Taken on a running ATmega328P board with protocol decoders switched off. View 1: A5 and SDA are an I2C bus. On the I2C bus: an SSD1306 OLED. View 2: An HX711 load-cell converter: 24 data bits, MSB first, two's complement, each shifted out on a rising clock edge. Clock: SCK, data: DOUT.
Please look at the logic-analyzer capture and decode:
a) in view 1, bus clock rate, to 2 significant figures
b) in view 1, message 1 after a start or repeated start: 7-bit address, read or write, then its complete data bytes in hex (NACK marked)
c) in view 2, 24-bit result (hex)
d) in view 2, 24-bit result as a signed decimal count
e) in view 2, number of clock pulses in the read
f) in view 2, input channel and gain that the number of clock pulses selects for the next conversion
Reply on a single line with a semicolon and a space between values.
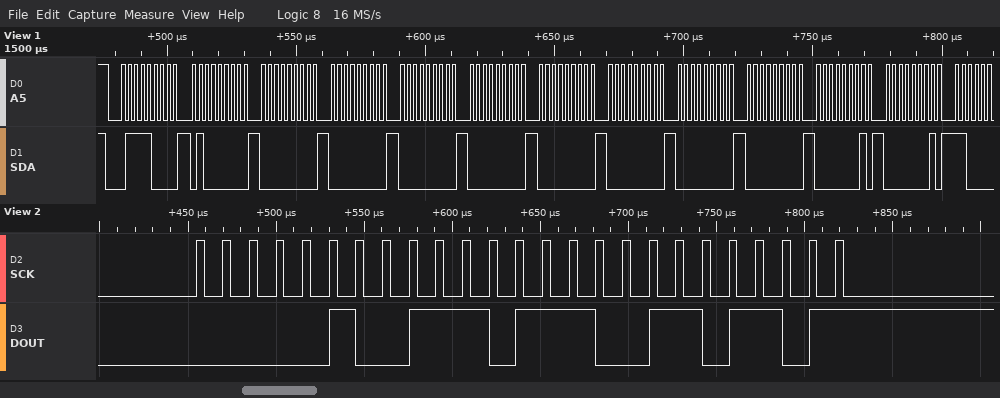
400 kHz; 0x3C write: 40 00 00 00 00 00 00 00 00 01 01; 0x04EE6D; 323181; 25; channel A, gain 128
